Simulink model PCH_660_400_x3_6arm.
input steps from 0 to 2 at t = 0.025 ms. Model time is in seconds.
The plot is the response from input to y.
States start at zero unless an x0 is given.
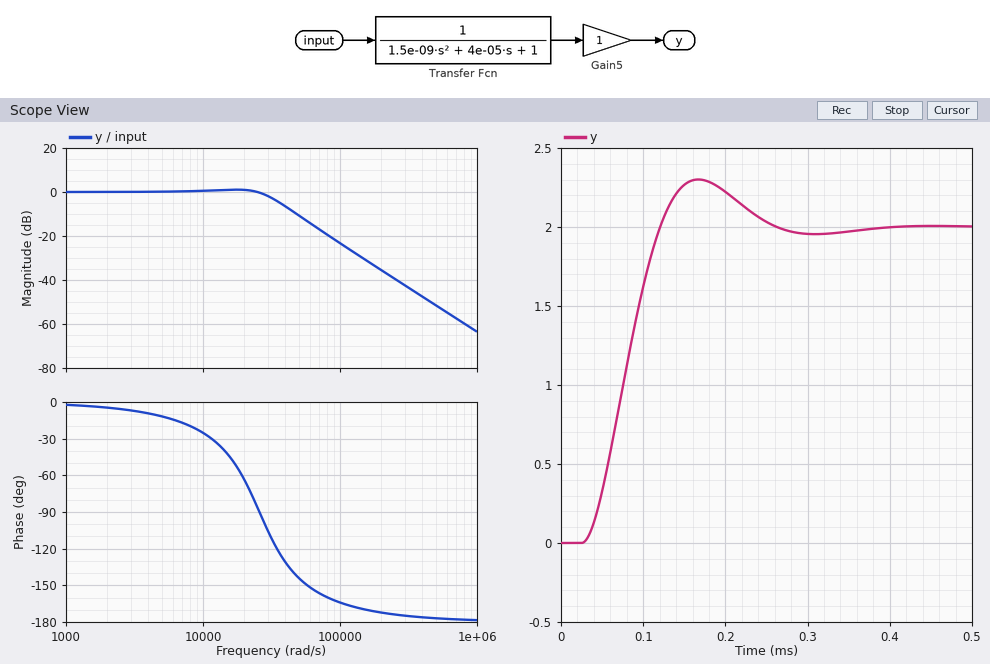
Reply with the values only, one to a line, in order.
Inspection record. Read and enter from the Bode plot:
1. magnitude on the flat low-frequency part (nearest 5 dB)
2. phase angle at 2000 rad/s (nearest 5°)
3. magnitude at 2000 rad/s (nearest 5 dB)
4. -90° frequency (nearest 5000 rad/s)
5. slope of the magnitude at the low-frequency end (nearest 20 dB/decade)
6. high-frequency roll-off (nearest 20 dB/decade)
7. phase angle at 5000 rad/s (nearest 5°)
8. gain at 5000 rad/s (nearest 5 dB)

0 dB
-5°
0 dB
25000 rad/s
0 dB/decade
-40 dB/decade
-10°
0 dB
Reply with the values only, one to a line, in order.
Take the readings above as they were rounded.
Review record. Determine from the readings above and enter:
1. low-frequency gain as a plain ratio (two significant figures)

1.0
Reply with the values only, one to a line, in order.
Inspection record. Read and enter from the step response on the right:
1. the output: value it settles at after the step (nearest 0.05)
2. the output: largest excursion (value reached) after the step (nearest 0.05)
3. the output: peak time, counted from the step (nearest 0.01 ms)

2.00
2.30
0.14 ms
